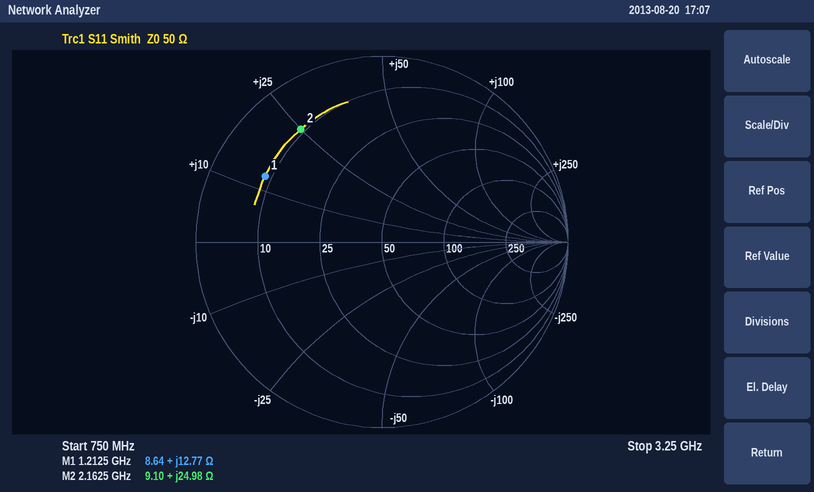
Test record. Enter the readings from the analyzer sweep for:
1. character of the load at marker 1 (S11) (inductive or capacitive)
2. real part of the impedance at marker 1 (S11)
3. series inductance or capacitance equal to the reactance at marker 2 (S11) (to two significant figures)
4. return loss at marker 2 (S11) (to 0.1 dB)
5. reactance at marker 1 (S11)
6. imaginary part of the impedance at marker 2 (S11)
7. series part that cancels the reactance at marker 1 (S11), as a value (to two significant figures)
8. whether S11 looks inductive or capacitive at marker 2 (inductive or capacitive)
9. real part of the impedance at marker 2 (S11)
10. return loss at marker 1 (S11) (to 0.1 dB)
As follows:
inductive
8.64 Ω
1.8 nH
2.5 dB
+12.77 Ω
+24.98 Ω
10 pF
inductive
9.10 Ω
2.8 dB
